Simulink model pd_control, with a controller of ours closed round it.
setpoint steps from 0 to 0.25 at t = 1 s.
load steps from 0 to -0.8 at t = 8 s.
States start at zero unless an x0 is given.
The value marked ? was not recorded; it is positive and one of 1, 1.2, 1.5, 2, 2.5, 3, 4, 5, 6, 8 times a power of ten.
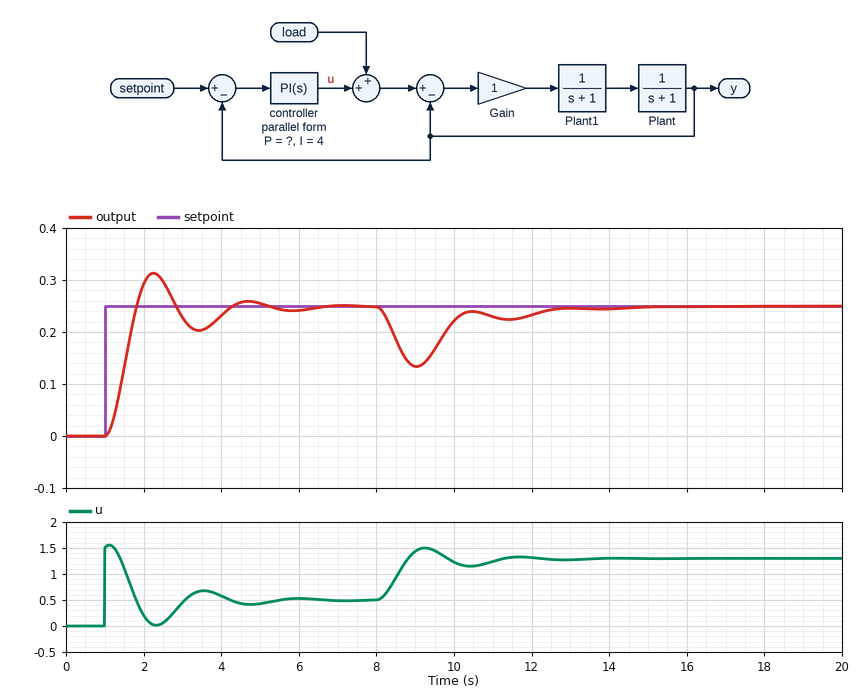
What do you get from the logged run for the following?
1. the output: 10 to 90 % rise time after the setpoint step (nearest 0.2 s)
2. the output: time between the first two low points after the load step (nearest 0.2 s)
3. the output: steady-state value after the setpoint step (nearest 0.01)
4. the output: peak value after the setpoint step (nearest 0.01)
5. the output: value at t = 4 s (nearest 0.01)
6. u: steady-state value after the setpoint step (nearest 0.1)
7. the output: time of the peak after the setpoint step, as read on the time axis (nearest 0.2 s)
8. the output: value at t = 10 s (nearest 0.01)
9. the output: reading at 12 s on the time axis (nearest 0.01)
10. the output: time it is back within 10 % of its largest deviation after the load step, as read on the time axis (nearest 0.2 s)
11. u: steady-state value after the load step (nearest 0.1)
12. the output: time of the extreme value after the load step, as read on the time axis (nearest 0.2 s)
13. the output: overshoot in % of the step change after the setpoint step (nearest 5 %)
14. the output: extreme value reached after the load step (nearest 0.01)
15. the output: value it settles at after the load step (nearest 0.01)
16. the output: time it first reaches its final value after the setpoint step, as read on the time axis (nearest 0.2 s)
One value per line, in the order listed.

0.6 s
2.4 s
0.25
0.31
0.23
0.5
2.2 s
0.22
0.23
12.2 s
1.3
9.0 s
25 %
0.13
0.25
1.8 s
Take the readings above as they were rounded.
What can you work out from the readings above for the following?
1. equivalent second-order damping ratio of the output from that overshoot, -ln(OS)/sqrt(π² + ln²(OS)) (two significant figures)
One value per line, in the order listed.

0.40
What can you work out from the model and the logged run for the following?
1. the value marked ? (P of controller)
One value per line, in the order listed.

6
